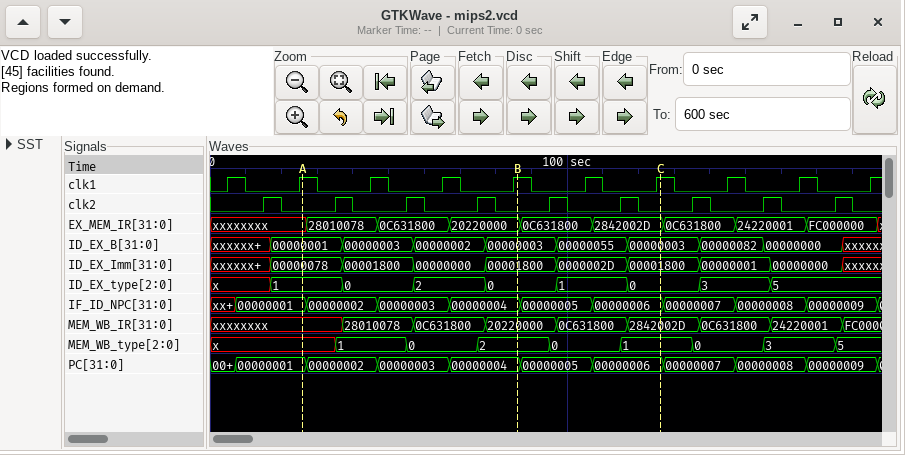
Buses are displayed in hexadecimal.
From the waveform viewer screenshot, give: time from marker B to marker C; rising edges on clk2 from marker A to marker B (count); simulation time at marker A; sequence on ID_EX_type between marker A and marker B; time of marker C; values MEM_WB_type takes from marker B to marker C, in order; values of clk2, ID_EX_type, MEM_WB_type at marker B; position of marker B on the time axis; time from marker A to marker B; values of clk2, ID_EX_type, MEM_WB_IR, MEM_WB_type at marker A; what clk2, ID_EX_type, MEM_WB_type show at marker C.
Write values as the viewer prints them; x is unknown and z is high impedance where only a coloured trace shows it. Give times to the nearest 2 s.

40 s
3
26 s
1, 0, 2, 0
126 s
2, 0, 1
clk2=0, ID_EX_type=0, MEM_WB_type=2
86 s
60 s
clk2=0, ID_EX_type=1, MEM_WB_IR=xxxxxxxx, MEM_WB_type=x
clk2=0, ID_EX_type=0, MEM_WB_type=1
